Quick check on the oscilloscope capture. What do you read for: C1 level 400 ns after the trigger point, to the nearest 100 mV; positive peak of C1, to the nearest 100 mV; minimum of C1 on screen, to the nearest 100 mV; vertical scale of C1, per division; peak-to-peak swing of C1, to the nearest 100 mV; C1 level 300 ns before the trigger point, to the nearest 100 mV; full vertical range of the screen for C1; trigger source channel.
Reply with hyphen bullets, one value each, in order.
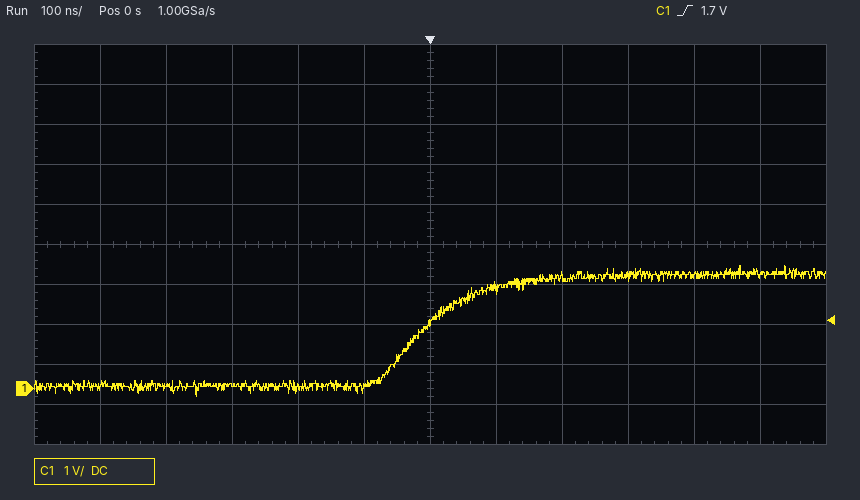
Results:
- 2.8 V
- 3.1 V
- -200 mV
- 1 V
- 3.3 V
- 100 mV
- 10 V
- C1
